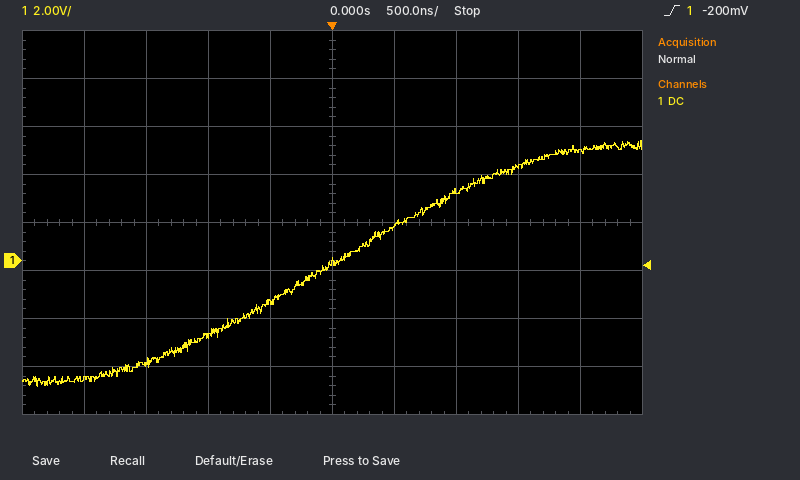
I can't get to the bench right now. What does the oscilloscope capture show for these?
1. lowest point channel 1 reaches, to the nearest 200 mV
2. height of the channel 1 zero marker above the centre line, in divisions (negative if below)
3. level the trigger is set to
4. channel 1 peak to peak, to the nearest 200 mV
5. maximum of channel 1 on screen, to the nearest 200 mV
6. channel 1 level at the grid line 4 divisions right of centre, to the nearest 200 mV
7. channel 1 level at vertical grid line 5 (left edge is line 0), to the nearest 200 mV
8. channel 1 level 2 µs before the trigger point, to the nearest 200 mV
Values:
-5.2 V
-0.8 div
-200 mV
10.2 V
5.0 V
4.6 V
0.0 V
-5.0 V
